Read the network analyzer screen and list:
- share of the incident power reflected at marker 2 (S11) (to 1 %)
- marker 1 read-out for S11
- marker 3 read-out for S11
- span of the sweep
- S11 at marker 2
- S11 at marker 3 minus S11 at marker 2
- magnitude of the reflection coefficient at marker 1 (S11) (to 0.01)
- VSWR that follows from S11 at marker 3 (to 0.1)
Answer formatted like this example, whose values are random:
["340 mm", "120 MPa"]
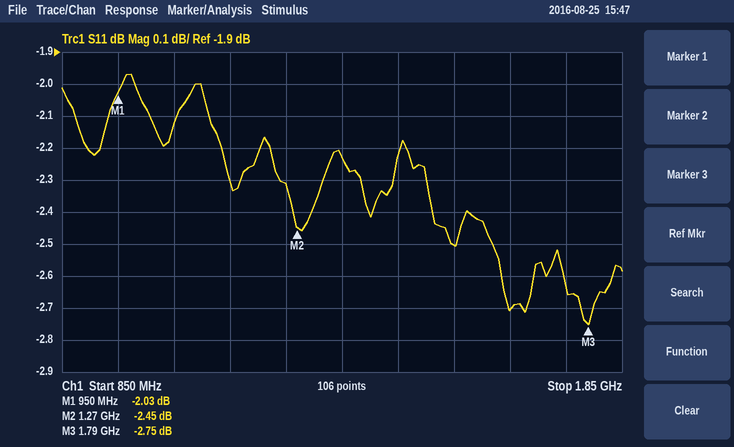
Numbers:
["57 %", "-2.03 dB", "-2.75 dB", "1 GHz", "-2.45 dB", "-0.30 dB", "0.79", "6.4"]
